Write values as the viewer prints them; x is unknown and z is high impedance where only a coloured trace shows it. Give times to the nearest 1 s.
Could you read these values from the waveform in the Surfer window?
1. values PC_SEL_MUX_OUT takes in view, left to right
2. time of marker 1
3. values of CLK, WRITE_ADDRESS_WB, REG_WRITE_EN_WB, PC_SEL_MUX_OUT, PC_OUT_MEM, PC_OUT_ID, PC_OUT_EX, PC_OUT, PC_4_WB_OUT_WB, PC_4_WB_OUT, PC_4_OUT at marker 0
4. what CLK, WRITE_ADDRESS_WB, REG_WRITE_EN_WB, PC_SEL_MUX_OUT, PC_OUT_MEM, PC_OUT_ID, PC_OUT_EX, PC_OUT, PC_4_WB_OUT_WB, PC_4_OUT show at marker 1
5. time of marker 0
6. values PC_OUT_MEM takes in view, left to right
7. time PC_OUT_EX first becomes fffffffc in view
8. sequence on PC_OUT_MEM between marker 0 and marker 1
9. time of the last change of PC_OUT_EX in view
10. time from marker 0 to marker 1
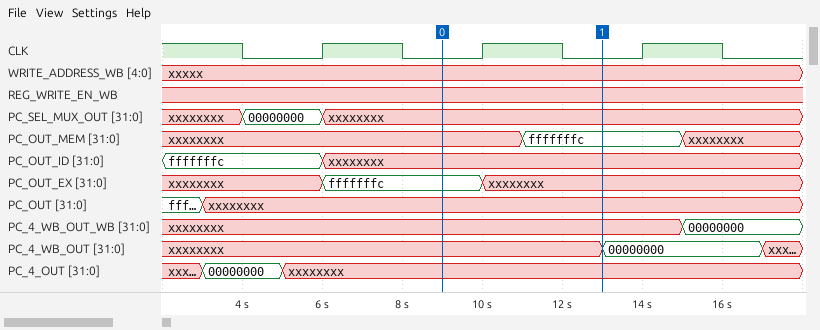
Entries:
xxxxxxxx, 00000000, xxxxxxxx
13 s
CLK=0, WRITE_ADDRESS_WB=xxxxx, REG_WRITE_EN_WB=x, PC_SEL_MUX_OUT=xxxxxxxx, PC_OUT_MEM=xxxxxxxx, PC_OUT_ID=xxxxxxxx, PC_OUT_EX=fffffffc, PC_OUT=xxxxxxxx, PC_4_WB_OUT_WB=xxxxxxxx, PC_4_WB_OUT=xxxxxxxx, PC_4_OUT=xxxxxxxx
CLK=0, WRITE_ADDRESS_WB=xxxxx, REG_WRITE_EN_WB=x, PC_SEL_MUX_OUT=xxxxxxxx, PC_OUT_MEM=fffffffc, PC_OUT_ID=xxxxxxxx, PC_OUT_EX=xxxxxxxx, PC_OUT=xxxxxxxx, PC_4_WB_OUT_WB=xxxxxxxx, PC_4_OUT=xxxxxxxx
9 s
xxxxxxxx, fffffffc, xxxxxxxx
6 s
xxxxxxxx, fffffffc
10 s
4 s
